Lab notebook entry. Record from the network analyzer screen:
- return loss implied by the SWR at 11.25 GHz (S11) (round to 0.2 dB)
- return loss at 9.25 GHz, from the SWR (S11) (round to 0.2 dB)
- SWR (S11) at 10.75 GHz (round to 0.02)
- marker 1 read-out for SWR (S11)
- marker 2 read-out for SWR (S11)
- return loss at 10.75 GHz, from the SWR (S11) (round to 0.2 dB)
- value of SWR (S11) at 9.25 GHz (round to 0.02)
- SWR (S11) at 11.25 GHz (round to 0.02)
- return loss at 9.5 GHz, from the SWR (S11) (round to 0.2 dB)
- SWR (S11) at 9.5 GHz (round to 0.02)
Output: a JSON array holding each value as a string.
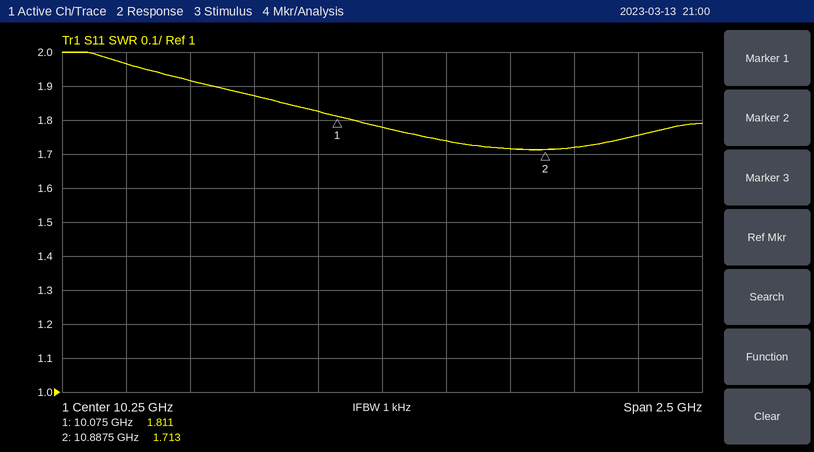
["11.2 dB", "9.8 dB", "1.72", "1.811", "1.713", "11.6 dB", "1.96", "1.76", "10.0 dB", "1.92"]
